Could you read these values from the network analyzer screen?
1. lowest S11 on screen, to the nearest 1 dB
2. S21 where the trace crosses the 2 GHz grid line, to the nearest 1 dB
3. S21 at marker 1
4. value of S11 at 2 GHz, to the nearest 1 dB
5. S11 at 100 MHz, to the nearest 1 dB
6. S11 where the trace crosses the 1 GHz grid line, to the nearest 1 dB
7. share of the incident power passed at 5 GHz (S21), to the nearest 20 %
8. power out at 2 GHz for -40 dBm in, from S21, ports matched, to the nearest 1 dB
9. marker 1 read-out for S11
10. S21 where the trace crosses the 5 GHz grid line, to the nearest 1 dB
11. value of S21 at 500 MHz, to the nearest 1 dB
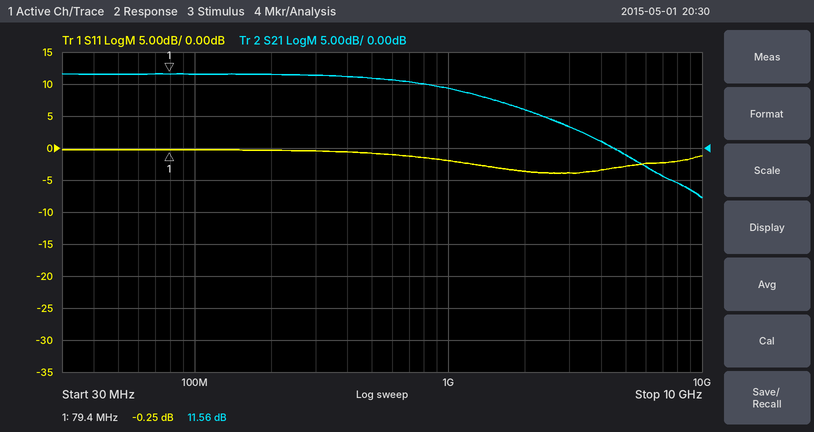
-4 dB
6 dB
11.56 dB
-4 dB
0 dB
-2 dB
80 %
-34 dBm
-0.25 dB
-1 dB
11 dB
